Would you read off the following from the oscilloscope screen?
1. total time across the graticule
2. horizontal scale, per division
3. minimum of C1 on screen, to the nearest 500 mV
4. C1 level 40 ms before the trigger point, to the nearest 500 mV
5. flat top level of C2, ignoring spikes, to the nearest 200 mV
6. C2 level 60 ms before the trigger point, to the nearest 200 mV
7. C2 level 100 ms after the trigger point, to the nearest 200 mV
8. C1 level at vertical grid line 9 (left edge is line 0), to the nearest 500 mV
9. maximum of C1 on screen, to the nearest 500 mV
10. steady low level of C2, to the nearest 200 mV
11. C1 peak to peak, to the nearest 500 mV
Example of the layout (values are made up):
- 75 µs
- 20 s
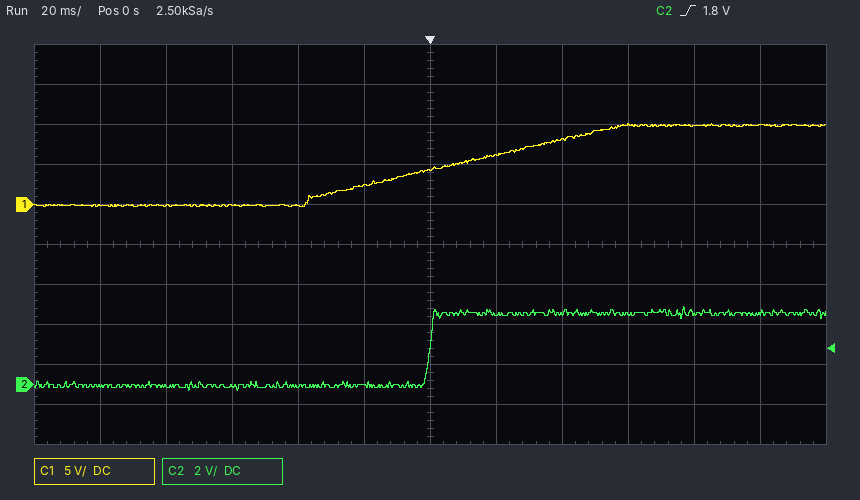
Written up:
- 240 ms
- 20 ms
- -500 mV
- 0.0 V
- 3.6 V
- 0.0 V
- 3.6 V
- 10.0 V
- 10.0 V
- 0.0 V
- 10.5 V
